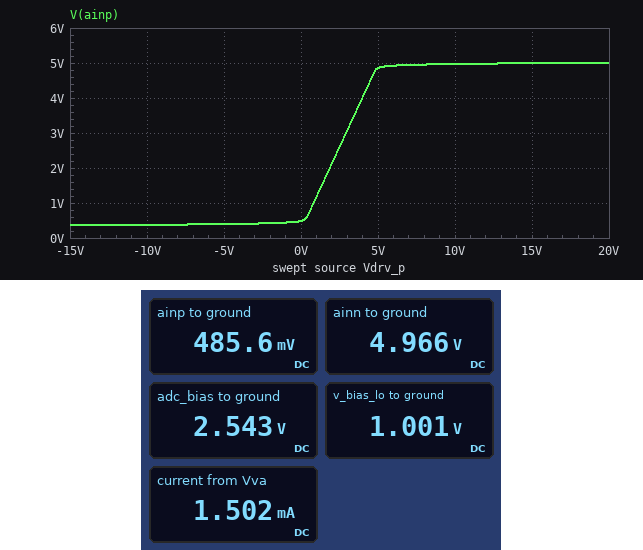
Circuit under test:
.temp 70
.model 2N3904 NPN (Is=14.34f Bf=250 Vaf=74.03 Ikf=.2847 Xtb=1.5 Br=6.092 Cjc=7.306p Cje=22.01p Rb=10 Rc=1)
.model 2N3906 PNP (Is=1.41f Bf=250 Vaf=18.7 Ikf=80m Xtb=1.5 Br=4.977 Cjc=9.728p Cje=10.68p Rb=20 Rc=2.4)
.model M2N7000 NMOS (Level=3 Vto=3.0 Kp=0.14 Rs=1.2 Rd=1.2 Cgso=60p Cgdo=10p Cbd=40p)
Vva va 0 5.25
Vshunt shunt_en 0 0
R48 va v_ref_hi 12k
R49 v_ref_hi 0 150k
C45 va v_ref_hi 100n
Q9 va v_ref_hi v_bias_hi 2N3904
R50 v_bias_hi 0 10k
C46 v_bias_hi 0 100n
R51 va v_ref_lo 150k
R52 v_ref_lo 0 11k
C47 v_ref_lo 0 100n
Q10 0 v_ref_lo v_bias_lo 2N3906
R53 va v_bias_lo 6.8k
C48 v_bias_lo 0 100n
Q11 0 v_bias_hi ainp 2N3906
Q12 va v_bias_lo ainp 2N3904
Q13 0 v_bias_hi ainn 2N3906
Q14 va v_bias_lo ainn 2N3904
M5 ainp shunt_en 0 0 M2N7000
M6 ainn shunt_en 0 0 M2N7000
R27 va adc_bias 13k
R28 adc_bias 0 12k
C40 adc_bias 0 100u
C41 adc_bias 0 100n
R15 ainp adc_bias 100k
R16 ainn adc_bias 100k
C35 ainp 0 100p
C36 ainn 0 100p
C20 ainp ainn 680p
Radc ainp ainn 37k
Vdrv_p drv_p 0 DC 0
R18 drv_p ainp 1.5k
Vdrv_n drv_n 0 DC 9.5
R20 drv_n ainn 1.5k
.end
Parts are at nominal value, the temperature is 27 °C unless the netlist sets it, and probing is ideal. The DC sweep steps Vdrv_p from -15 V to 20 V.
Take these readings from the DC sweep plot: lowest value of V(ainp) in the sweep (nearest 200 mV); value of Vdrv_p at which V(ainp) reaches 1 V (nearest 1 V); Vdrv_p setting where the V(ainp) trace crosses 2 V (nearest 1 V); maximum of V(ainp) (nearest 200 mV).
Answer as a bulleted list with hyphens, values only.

- 400 mV
- 1 V
- 2 V
- 5.0 V
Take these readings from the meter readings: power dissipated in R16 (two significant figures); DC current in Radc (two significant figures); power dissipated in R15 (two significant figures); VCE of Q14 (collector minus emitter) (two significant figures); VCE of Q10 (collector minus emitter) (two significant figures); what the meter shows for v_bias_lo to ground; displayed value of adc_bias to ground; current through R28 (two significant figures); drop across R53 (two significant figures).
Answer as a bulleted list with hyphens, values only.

- 59 µW
- 120 µA
- 42 µW
- 280 mV
- -1.0 V
- 1.001 V
- 2.543 V
- 210 µA
- 4.2 V
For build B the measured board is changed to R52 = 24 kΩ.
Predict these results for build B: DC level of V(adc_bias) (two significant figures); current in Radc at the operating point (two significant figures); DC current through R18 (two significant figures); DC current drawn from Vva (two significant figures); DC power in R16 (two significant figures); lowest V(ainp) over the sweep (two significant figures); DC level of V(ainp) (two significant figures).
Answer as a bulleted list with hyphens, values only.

- 2.6 V
- 110 µA
- 560 µA
- 1.7 mA
- 58 µW
- 740 mV
- 840 mV
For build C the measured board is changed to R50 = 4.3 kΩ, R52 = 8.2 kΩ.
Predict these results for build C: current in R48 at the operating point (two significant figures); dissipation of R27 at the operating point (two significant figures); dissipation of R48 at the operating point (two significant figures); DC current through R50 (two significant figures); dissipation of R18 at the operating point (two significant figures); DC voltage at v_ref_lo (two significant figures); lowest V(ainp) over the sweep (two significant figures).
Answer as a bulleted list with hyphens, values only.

- 35 µA
- 570 µW
- 15 µW
- 990 µA
- 110 µW
- 290 mV
- 270 mV
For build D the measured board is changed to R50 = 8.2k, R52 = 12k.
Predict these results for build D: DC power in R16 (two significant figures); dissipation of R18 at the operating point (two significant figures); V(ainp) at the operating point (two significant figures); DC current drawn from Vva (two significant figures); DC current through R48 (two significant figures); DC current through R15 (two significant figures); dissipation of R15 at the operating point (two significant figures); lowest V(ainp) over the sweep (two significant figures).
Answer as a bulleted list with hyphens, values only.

- 58 µW
- 180 µW
- 510 mV
- 1.6 mA
- 34 µA
- 20 µA
- 41 µW
- 390 mV
